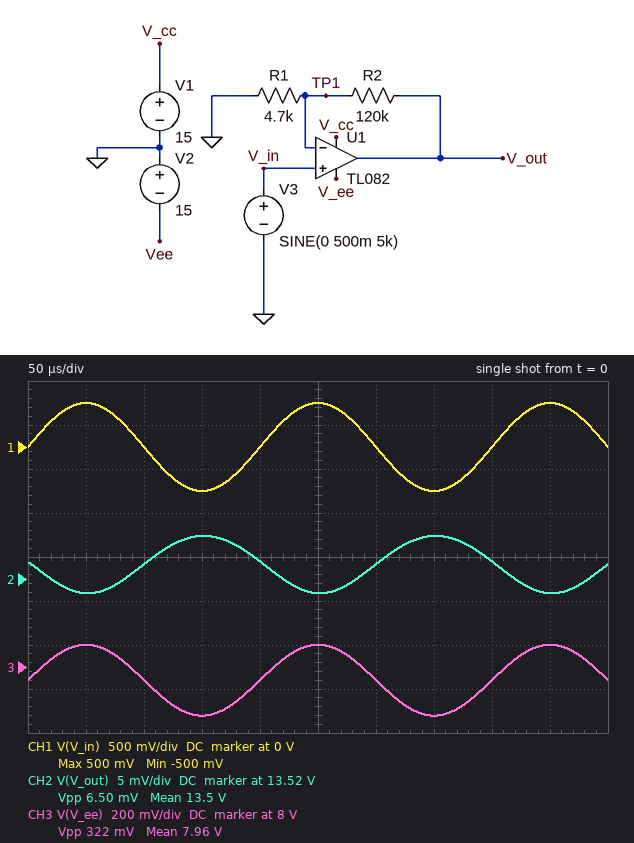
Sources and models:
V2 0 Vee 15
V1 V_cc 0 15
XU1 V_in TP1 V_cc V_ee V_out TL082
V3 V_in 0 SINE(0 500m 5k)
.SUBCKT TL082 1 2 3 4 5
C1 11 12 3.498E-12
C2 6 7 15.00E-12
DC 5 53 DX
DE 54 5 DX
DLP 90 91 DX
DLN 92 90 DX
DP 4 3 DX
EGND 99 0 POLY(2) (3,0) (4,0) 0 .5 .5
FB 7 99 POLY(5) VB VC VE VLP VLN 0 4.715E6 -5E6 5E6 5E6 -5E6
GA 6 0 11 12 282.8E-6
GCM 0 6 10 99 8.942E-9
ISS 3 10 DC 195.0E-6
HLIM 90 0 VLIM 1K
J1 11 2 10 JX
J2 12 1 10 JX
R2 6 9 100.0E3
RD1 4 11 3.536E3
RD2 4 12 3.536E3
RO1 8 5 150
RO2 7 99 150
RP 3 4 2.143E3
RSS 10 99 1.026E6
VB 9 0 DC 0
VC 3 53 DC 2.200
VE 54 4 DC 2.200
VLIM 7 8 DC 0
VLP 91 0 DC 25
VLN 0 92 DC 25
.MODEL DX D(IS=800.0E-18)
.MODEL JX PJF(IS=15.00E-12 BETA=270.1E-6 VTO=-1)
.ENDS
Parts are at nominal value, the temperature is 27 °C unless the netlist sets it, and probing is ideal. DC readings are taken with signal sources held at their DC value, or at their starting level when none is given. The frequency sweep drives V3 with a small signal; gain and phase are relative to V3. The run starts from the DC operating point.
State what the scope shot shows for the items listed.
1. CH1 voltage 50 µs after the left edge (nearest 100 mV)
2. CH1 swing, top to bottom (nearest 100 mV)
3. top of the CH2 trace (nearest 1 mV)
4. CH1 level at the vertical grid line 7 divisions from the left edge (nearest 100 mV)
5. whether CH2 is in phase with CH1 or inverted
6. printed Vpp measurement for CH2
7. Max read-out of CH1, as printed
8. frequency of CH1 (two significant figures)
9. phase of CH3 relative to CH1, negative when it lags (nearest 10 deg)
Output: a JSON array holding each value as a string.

["500 mV", "1.0 V", "13.520 V", "-500 mV", "inverted", "6.50 mV", "500 mV", "5.0 kHz", "0 deg"]
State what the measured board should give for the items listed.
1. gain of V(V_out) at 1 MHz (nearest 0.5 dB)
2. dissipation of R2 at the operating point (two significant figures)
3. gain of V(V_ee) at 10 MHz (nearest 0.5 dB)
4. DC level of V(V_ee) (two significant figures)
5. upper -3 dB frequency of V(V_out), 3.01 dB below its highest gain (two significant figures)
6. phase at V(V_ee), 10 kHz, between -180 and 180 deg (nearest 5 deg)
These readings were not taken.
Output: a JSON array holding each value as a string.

["-63.5 dB", "870 µW", "-8.5 dB", "7.9 V", "110 kHz", "0 deg"]
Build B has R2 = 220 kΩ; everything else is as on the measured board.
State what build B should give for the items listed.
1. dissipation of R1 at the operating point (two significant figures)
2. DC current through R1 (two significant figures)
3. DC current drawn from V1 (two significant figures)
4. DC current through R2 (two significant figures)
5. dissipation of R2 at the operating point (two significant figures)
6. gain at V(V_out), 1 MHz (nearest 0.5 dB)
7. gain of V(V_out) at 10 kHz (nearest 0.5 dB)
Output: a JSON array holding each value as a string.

["2.2 mW", "680 µA", "2.7 mA", "47 µA", "480 µW", "-63.0 dB", "-43.5 dB"]
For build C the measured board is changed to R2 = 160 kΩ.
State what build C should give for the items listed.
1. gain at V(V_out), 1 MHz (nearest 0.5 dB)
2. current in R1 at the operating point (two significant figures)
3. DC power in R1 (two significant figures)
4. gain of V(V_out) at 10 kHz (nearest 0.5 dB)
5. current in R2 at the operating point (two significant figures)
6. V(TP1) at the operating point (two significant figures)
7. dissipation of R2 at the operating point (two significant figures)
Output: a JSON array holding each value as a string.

["-63.0 dB", "690 µA", "2.2 mW", "-43.5 dB", "64 µA", "3.2 V", "660 µW"]
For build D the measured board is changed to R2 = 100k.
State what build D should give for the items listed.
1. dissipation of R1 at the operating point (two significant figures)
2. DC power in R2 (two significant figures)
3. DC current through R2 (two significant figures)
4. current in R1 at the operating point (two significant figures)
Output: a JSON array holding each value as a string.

["2.4 mW", "1.0 mW", "100 µA", "710 µA"]
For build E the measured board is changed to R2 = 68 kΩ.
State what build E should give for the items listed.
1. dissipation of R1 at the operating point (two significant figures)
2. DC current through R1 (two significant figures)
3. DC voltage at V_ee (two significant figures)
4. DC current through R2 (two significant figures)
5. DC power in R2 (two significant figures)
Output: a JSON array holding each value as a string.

["2.5 mW", "730 µA", "8.0 V", "150 µA", "1.5 mW"]
